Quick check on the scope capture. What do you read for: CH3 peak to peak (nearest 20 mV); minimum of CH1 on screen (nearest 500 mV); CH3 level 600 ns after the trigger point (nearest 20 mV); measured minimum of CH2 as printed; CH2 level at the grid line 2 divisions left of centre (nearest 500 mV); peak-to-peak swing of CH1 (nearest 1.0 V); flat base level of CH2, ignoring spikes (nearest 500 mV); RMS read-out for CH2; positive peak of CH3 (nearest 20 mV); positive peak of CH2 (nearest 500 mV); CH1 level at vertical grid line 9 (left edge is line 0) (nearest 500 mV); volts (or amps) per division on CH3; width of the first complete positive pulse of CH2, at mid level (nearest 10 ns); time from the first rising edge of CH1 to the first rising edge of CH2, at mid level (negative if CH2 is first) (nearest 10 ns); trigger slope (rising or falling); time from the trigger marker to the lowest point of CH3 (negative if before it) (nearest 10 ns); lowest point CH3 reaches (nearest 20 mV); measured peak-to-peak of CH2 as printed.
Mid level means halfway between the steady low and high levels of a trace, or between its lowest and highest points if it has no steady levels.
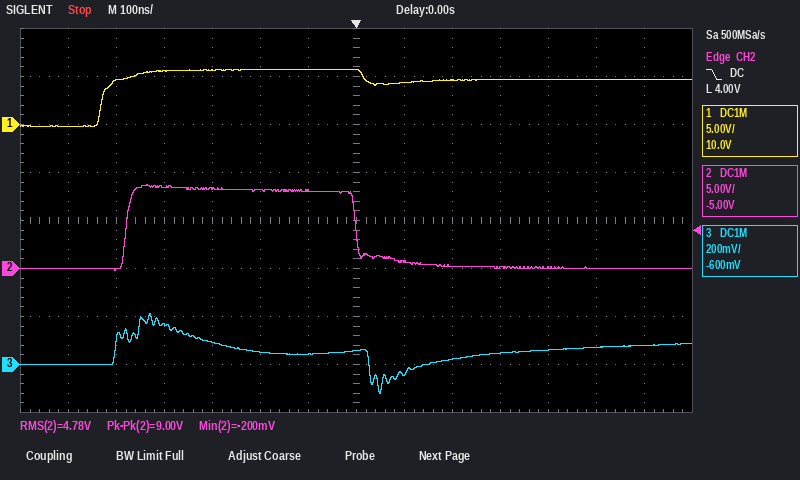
340 mV
0.0 V
80 mV
-200 mV
8.0 V
6.0 V
0.0 V
4.78 V
220 mV
9.0 V
4.5 V
200 mV
480 ns
+50 ns
falling
+50 ns
-120 mV
9.00 V
